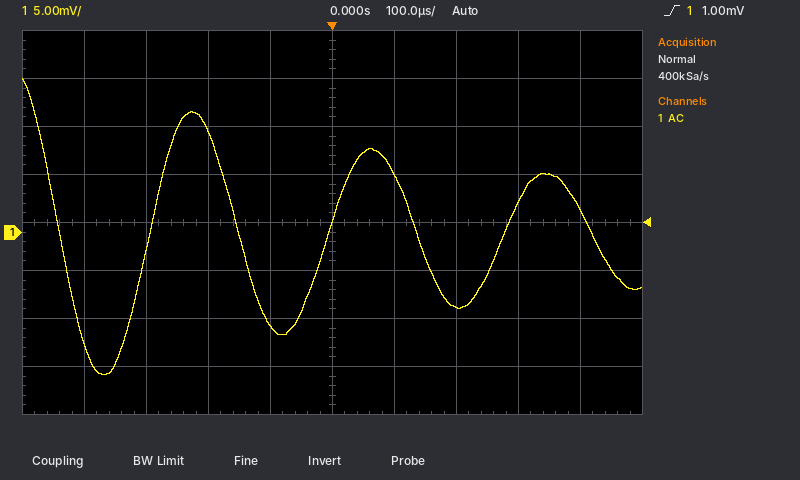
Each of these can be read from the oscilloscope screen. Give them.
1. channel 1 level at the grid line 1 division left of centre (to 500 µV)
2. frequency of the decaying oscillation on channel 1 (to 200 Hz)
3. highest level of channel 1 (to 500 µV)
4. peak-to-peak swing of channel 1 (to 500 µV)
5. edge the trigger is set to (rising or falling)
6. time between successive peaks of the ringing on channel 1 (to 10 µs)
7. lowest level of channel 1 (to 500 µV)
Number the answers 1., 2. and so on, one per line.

1. -9.5 mV
2. 3.6 kHz
3. 16.0 mV
4. 31.0 mV
5. rising
6. 280 µs
7. -15.0 mV
